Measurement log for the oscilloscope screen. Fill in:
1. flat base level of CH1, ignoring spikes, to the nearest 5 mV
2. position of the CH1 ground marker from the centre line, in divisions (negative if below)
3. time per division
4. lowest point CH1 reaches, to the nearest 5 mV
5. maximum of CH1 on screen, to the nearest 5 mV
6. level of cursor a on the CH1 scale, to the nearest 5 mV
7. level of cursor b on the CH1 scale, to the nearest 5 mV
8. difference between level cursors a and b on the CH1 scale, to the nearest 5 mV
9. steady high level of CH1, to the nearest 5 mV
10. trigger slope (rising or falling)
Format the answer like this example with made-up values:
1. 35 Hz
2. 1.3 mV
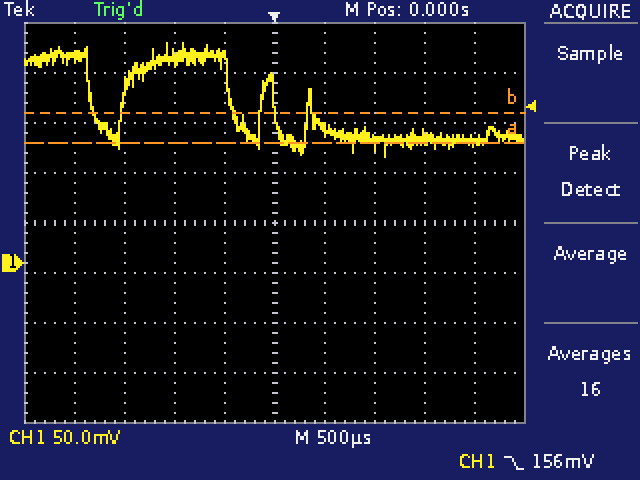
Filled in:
1. 125 mV
2. -0.8 div
3. 500 µs
4. 105 mV
5. 220 mV
6. 120 mV
7. 150 mV
8. 30 mV
9. 205 mV
10. falling
